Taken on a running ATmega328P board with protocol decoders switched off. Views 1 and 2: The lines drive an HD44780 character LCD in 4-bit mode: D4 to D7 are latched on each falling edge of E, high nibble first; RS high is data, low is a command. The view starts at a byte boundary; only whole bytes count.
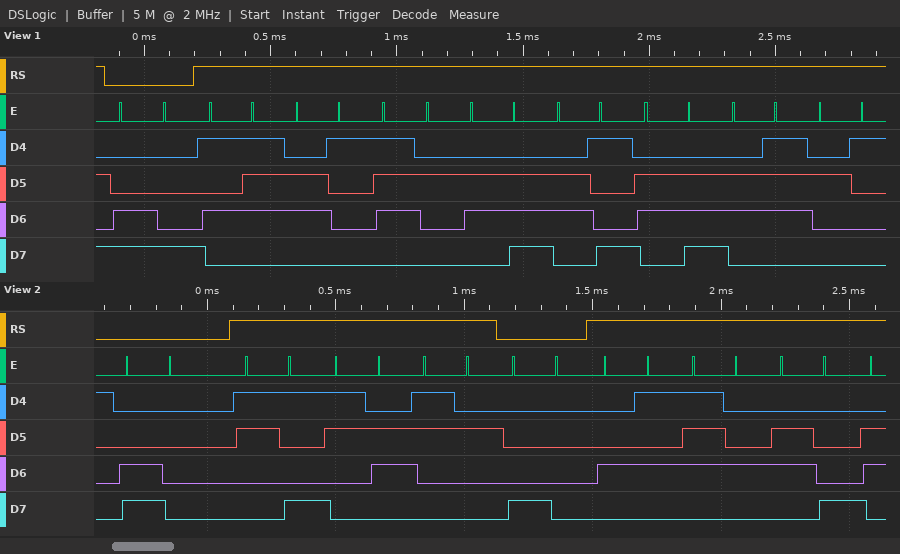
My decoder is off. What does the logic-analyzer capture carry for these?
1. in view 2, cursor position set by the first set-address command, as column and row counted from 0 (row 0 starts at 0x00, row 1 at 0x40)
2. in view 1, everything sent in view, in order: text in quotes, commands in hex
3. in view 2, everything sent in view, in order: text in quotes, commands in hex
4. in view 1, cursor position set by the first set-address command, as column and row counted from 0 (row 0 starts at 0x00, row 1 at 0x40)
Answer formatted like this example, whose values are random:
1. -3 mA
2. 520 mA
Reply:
1. column 0, row 1
2. 0xC8 "Warning!"
3. 0xC0 "962" 0x80 "Eth"
4. column 8, row 1
